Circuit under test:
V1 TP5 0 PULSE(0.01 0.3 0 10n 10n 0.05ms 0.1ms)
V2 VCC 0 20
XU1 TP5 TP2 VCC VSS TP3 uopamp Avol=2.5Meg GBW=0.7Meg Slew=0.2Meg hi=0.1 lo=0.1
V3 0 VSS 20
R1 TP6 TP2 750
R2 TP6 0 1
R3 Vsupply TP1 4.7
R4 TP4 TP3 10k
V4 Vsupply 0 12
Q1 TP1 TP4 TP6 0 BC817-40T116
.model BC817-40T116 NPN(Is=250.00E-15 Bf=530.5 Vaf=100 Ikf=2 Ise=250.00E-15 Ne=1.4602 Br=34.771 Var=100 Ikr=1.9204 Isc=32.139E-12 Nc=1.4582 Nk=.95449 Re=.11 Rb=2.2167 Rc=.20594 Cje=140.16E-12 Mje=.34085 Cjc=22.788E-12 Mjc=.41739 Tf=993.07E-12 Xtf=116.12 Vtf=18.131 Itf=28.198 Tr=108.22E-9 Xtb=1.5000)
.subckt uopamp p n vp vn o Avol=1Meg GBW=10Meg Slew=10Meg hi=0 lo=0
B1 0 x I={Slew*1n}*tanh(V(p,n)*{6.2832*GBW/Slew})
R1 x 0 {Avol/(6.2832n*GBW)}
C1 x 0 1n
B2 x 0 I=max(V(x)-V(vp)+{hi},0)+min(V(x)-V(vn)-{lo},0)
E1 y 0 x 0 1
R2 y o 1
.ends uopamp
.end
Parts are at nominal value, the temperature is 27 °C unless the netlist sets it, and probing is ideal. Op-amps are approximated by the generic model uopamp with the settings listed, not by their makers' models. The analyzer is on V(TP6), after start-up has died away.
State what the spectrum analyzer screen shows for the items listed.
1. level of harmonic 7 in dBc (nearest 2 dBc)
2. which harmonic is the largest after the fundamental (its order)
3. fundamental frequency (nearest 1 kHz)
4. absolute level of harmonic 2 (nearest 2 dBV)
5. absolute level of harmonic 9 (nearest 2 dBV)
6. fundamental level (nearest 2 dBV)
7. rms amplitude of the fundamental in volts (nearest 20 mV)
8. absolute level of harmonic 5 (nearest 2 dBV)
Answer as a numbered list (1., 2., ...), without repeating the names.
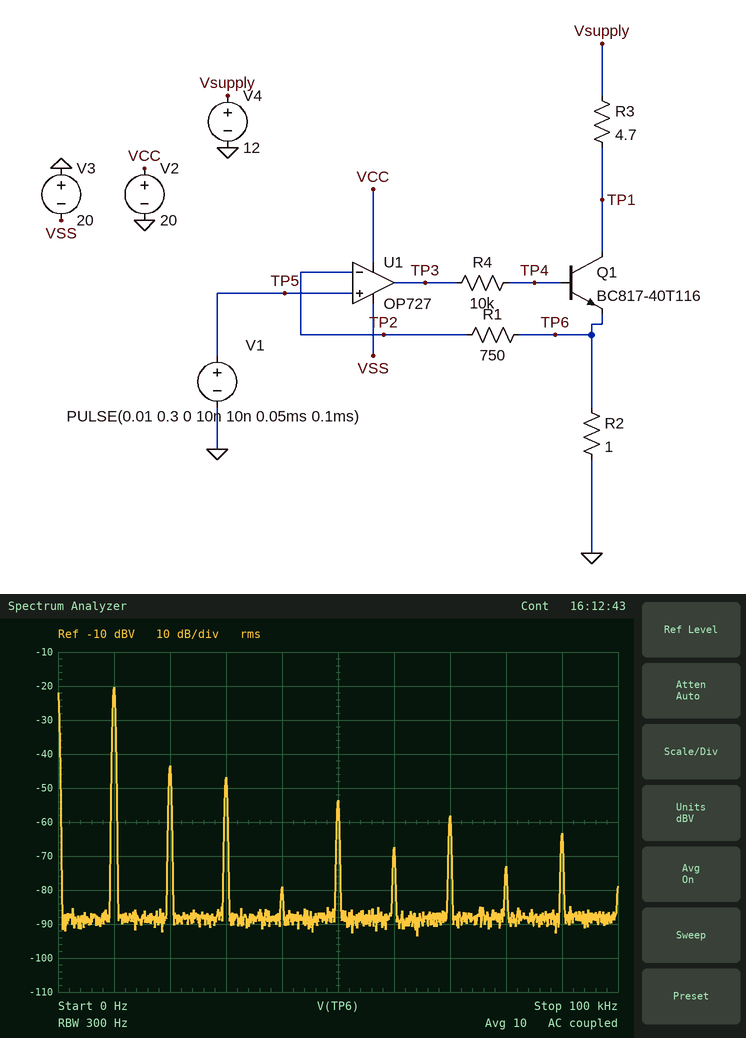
1. -38 dBc
2. 2
3. 10 kHz
4. -44 dBV
5. -64 dBV
6. -20 dBV
7. 100 mV
8. -54 dBV
